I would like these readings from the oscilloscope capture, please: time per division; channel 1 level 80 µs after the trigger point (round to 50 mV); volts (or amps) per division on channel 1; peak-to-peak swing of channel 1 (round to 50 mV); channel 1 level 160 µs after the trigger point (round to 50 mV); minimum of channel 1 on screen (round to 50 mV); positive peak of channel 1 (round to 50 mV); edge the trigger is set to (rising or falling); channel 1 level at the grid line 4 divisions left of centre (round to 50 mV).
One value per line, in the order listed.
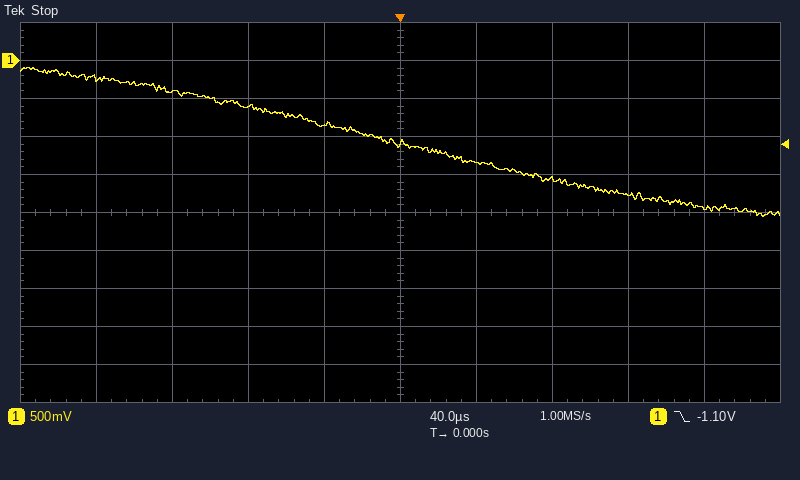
40 µs
-1.55 V
500 mV
1.95 V
-1.95 V
-2.05 V
-100 mV
falling
-250 mV
